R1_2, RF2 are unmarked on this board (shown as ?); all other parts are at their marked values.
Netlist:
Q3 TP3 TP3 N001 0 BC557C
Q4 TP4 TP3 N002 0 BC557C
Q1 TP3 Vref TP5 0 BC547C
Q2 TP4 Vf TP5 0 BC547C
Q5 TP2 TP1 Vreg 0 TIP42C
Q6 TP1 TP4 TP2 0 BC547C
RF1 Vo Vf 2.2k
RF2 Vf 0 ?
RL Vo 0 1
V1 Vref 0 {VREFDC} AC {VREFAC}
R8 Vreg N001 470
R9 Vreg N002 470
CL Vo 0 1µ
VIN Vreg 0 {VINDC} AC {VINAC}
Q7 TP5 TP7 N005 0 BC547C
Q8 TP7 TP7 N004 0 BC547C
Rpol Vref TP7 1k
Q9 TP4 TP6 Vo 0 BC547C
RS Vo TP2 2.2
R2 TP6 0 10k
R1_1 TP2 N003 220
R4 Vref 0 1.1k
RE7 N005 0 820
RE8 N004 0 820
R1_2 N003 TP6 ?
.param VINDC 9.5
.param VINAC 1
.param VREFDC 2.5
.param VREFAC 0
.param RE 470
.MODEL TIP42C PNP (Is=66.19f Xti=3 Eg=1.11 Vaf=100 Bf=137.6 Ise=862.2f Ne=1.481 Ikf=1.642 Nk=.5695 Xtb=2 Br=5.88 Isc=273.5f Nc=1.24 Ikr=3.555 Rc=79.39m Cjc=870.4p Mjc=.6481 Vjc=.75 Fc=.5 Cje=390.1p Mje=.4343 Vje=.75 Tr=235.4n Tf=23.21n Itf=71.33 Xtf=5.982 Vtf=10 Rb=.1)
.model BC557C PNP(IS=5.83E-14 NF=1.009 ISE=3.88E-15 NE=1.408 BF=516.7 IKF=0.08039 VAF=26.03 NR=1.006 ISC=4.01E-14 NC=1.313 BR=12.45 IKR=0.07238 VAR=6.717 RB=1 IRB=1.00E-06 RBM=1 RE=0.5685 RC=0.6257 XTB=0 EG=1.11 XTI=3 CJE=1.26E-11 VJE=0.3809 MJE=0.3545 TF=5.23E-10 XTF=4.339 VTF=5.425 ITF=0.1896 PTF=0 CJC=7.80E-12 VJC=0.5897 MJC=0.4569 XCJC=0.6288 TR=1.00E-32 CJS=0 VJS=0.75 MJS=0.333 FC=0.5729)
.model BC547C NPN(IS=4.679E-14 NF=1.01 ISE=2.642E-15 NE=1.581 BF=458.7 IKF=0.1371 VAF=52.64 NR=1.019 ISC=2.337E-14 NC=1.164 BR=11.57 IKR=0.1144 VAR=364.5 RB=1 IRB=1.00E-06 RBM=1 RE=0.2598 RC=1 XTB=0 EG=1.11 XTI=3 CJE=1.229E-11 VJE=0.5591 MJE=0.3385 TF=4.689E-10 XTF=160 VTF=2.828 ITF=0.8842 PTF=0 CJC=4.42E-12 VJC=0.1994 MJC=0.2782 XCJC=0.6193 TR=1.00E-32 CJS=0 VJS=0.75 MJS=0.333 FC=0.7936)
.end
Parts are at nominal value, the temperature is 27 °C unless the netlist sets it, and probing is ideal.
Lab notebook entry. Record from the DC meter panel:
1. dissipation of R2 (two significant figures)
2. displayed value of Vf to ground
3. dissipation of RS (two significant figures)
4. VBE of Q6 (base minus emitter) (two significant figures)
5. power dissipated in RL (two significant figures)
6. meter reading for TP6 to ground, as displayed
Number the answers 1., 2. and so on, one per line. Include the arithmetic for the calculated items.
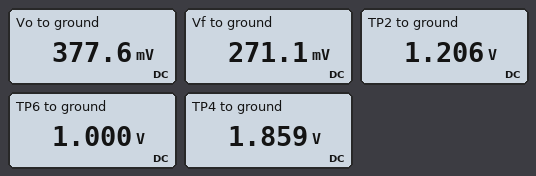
1. (1 V)^2 / 10 kΩ = 100 µW
2. 271.1 mV
3. (1.206 V - 377.6 mV)^2 / 2.2 Ω = 310 mW
4. 1.859 V - 1.206 V = 650 mV
5. (377.6 mV)^2 / 1 Ω = 140 mW
6. 1.000 V
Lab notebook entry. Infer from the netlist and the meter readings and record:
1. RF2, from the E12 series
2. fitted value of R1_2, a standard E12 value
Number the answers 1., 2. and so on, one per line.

1. 5.6 kΩ
2. 1.8 kΩ
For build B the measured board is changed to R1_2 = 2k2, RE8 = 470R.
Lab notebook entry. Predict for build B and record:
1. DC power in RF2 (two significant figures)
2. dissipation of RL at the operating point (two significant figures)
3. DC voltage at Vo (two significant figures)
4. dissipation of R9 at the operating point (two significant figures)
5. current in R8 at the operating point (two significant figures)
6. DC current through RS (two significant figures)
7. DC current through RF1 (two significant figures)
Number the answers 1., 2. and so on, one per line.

1. 14 µW
2. 150 mW
3. 390 mV
4. 270 µW
5. 740 µA
6. 390 mA
7. 50 µA
